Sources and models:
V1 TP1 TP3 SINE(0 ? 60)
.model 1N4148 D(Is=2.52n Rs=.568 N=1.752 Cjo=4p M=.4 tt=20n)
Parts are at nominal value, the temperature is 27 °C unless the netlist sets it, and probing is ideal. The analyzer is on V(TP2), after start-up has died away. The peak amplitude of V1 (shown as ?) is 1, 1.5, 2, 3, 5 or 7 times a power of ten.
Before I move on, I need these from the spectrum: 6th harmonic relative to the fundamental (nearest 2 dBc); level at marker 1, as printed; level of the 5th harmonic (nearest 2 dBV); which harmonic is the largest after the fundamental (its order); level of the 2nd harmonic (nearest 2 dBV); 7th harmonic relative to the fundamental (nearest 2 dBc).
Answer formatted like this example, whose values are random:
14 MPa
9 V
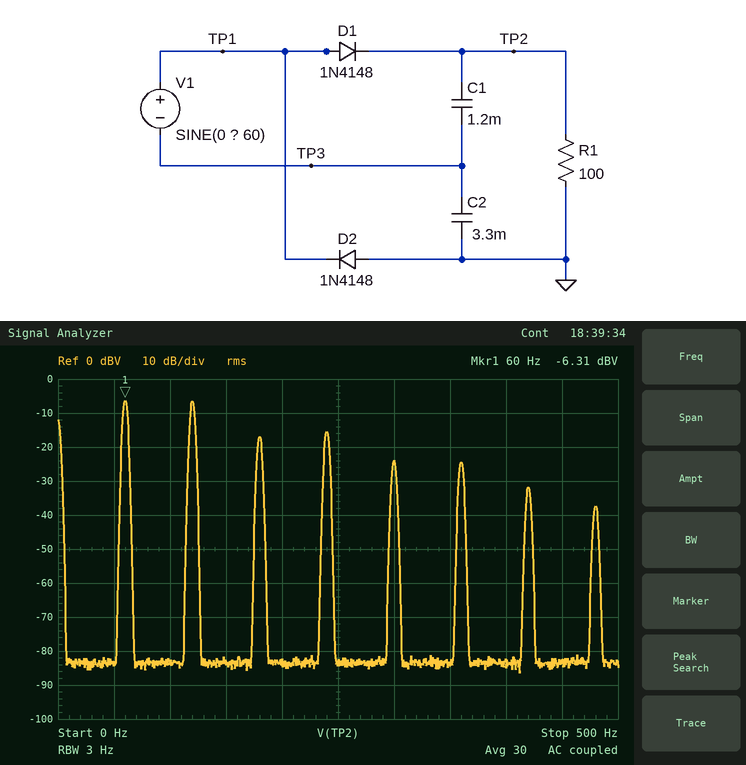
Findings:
-18 dBc
-6.31 dBV
-24 dBV
2
-6 dBV
-26 dBc
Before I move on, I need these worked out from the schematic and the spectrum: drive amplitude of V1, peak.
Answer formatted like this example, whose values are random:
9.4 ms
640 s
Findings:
15 V
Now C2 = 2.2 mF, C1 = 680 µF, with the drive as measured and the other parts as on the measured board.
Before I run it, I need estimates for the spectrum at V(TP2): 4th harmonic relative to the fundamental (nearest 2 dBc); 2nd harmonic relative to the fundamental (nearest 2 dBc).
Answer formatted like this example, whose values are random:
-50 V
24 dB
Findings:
-12 dBc
-2 dBc
